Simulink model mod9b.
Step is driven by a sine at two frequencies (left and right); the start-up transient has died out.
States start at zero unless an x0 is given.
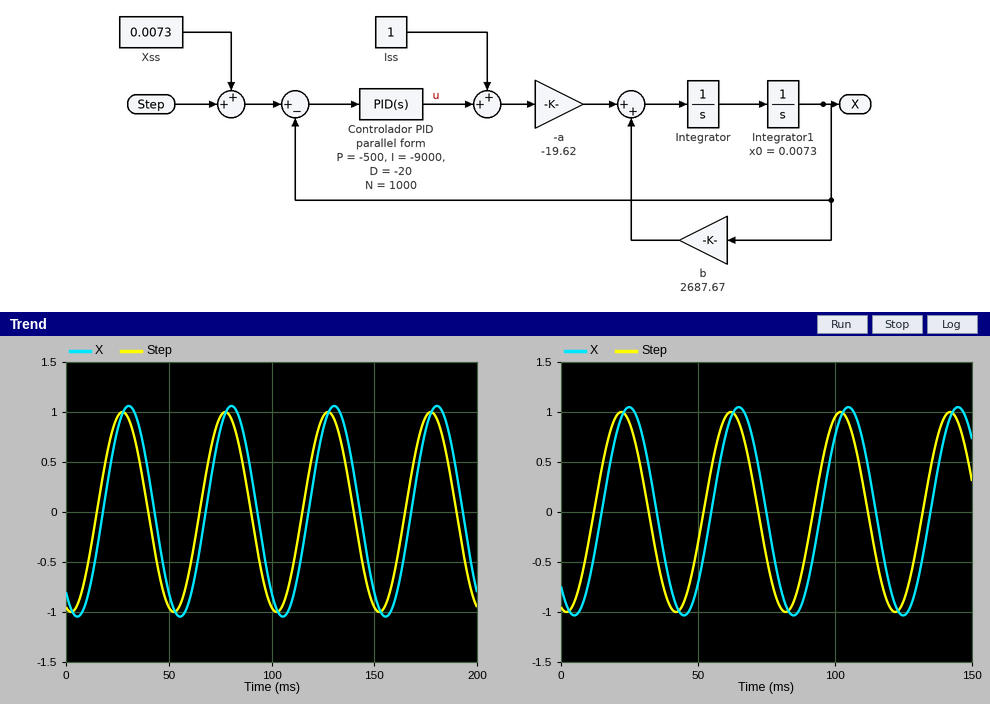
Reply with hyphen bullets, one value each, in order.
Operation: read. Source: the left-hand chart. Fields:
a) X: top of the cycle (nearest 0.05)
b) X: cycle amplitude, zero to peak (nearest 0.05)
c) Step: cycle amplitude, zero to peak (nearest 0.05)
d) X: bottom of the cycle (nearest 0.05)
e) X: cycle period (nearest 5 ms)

- 1.05
- 1.05
- 1.00
- -1.05
- 50 ms
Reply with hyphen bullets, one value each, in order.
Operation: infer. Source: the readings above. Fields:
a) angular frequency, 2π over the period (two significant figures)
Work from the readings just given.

- 0.13 rad/ms
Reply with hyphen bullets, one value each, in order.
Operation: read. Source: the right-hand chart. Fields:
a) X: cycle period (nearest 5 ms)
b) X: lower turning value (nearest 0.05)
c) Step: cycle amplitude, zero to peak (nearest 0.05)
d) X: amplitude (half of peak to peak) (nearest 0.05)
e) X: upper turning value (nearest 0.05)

- 40 ms
- -1.05
- 1.00
- 1.05
- 1.05
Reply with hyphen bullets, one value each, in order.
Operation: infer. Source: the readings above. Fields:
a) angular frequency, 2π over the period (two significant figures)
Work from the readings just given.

- 0.16 rad/ms
